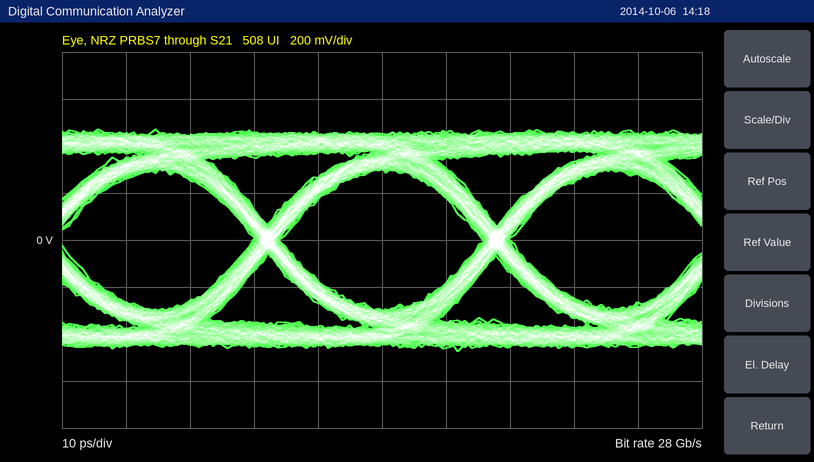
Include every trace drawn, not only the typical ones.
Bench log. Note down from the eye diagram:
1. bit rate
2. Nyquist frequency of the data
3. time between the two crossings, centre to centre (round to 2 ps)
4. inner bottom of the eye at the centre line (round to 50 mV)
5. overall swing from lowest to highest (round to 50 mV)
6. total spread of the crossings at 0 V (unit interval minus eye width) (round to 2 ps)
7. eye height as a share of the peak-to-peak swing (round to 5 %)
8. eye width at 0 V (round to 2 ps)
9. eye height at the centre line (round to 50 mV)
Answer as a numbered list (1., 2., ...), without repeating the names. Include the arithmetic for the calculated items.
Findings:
1. 28 Gb/s
2. 14 GHz
3. 36 ps
4. -300 mV
5. 950 mV
6. 4 ps
7. 600 mV / 950 mV ≈ 63.2 %, so 65 % to the nearest 5 %
8. 32 ps
9. 600 mV
